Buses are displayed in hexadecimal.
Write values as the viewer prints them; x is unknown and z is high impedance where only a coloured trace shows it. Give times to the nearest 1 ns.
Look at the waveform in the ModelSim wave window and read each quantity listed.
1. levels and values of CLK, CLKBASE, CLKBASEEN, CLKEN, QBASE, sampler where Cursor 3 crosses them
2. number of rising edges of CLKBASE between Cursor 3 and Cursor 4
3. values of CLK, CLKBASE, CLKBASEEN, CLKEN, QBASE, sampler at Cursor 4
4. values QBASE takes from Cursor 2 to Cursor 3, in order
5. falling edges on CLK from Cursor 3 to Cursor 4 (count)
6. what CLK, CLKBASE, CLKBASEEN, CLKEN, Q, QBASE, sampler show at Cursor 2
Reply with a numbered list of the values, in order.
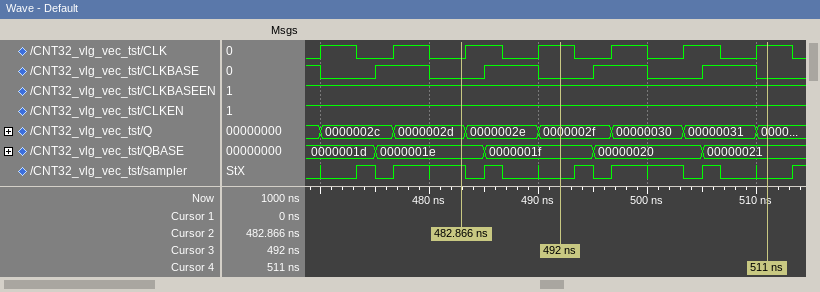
1. CLK=1, CLKBASE=0, CLKBASEEN=1, CLKEN=1, QBASE=0000001f, sampler=0
2. 2
3. CLK=1, CLKBASE=0, CLKBASEEN=1, CLKEN=1, QBASE=00000021, sampler=0
4. 0000001e, 0000001f
5. 3
6. CLK=0, CLKBASE=0, CLKBASEEN=1, CLKEN=1, Q=0000002d, QBASE=0000001e, sampler=1
